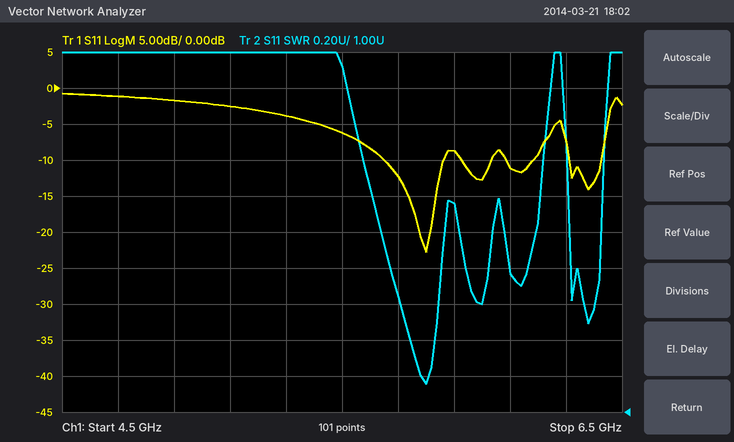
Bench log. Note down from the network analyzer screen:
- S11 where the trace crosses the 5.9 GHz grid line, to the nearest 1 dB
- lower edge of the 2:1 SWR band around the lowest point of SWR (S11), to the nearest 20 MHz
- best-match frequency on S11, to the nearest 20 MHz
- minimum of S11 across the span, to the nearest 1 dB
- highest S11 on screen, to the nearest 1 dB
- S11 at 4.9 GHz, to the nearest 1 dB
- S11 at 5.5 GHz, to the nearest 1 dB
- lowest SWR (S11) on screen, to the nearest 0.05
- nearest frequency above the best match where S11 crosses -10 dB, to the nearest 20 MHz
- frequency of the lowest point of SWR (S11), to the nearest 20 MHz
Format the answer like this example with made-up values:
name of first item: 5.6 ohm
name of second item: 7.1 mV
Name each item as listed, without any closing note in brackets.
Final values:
S11 where the trace crosses the 5.9 GHz grid line, to the nearest 1 dB: -9 dB
lower edge of the 2:1 SWR band around the lowest point of SWR (S11), to the nearest 20 MHz: 5.64 GHz
best-match frequency on S11, to the nearest 20 MHz: 5.80 GHz
minimum of S11 across the span, to the nearest 1 dB: -23 dB
highest S11 on screen, to the nearest 1 dB: -1 dB
S11 at 4.9 GHz, to the nearest 1 dB: -2 dB
S11 at 5.5 GHz, to the nearest 1 dB: -6 dB
lowest SWR (S11) on screen, to the nearest 0.05: 1.15
nearest frequency above the best match where S11 crosses -10 dB, to the nearest 20 MHz: 5.86 GHz
frequency of the lowest point of SWR (S11), to the nearest 20 MHz: 5.80 GHz
